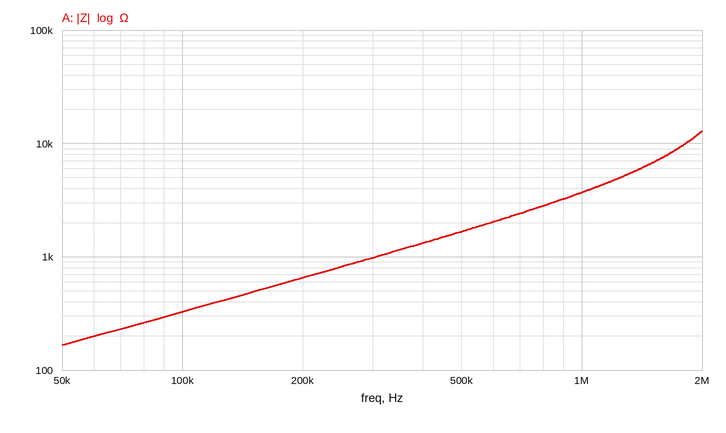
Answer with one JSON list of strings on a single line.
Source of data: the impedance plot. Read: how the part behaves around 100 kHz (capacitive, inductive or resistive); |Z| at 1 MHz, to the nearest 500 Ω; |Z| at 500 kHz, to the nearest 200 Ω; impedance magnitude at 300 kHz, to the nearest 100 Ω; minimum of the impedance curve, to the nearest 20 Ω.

["inductive", "3.5 kΩ", "1.6 kΩ", "1.0 kΩ", "160 Ω"]
